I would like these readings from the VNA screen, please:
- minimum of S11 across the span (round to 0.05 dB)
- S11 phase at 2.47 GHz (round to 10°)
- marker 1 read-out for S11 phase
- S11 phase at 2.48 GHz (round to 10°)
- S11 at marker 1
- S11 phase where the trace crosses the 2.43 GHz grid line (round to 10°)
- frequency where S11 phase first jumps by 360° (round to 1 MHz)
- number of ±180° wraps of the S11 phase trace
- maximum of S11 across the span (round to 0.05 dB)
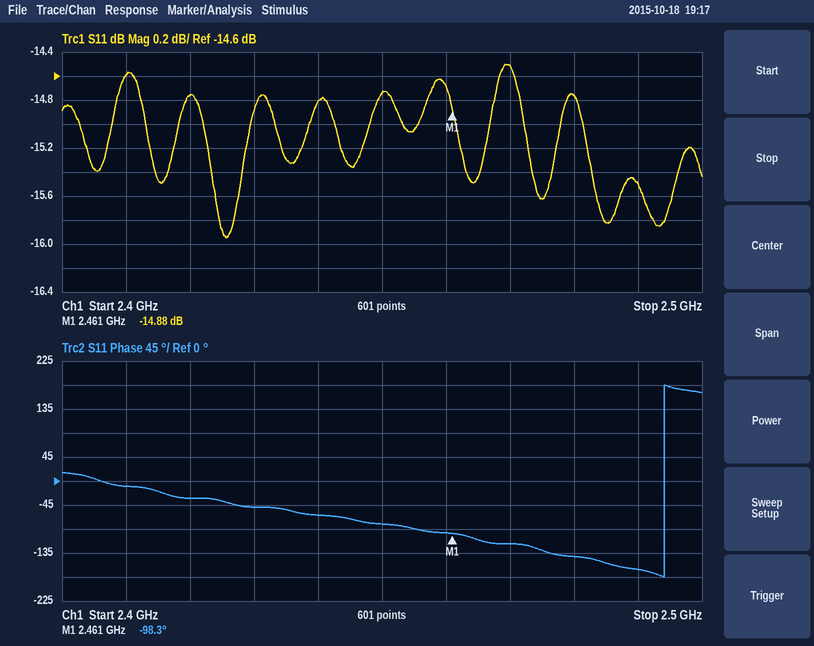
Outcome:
-15.95 dB
-120°
-98.3°
-140°
-14.88 dB
-50°
2.494 GHz
1
-14.50 dB
